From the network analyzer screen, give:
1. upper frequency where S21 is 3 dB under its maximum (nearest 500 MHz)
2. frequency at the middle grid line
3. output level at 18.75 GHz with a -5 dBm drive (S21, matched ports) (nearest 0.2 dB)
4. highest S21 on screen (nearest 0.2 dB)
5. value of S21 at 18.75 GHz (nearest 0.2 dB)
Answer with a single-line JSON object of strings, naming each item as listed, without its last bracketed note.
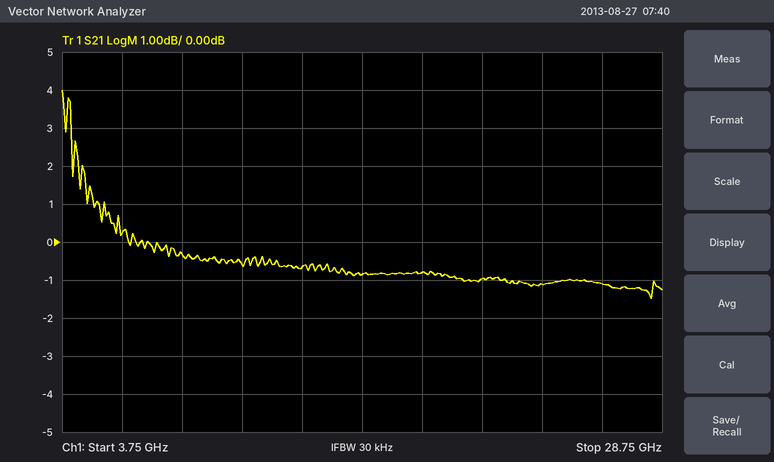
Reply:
{"upper frequency where S21 is 3 dB under its maximum": "5.0 GHz", "frequency at the middle grid line": "16.25 GHz", "output level at 18.75 GHz with a -5 dBm drive (S21, matched ports)": "-5.8 dBm", "highest S21 on screen": "4.0 dB", "value of S21 at 18.75 GHz": "-0.8 dB"}
